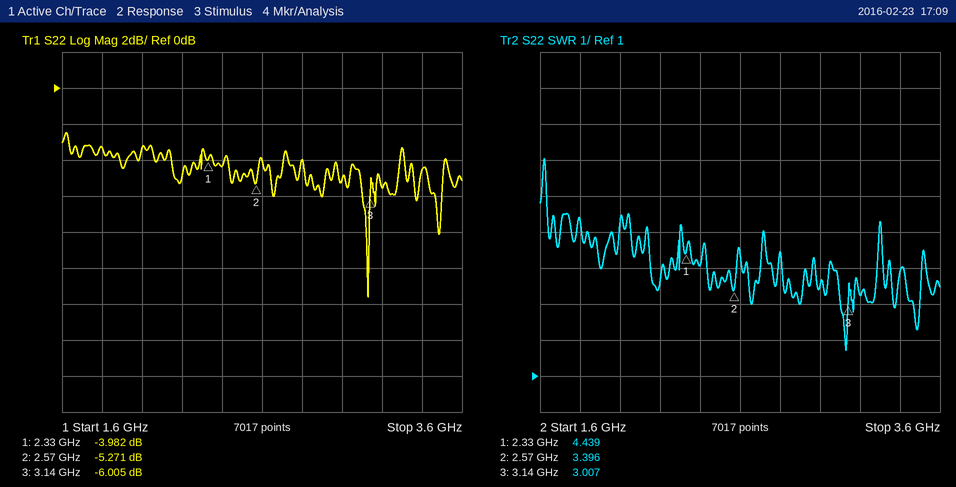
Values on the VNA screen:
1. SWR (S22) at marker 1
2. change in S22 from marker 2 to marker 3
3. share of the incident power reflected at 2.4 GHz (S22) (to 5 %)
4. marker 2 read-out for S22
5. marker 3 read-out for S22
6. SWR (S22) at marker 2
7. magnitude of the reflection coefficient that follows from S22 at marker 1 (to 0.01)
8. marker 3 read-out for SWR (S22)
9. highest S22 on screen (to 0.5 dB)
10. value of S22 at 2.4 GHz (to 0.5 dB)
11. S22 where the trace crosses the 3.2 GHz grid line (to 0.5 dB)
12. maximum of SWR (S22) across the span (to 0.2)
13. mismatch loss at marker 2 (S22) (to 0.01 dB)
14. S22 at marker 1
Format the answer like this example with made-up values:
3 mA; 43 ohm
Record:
4.439; -0.734 dB; 35 %; -5.271 dB; -6.005 dB; 3.396; 0.63; 3.007; -2.5 dB; -4.5 dB; -5.5 dB; 7.0; 1.53 dB; -3.982 dB
